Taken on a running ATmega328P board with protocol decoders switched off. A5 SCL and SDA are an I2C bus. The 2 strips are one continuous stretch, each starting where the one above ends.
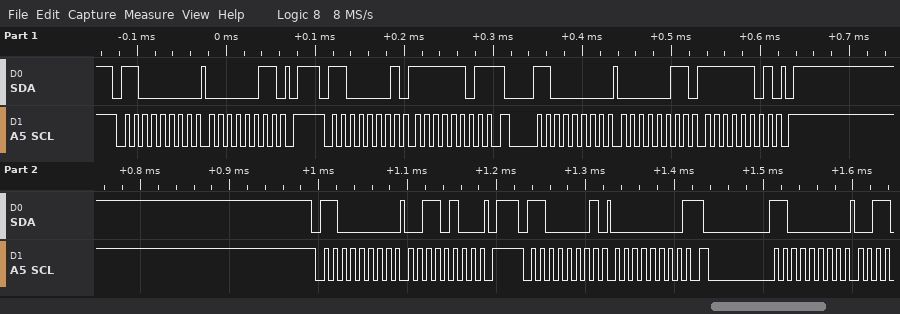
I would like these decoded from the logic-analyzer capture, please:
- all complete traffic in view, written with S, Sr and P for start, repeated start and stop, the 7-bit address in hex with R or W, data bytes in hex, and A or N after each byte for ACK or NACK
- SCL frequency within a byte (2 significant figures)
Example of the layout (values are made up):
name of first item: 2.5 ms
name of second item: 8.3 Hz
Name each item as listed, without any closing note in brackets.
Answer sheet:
all complete traffic in view, written with S, Sr and P for start, repeated start and stop, the 7-bit address in hex with R or W, data bytes in hex, and A or N after each byte for ACK or NACK: S 60W A 03 A P S 60R A FD N Sr 60W A 03 A FD A P S 60W A 34 A P S 60R A 00 N Sr 60W A
SCL frequency within a byte: 100 kHz
